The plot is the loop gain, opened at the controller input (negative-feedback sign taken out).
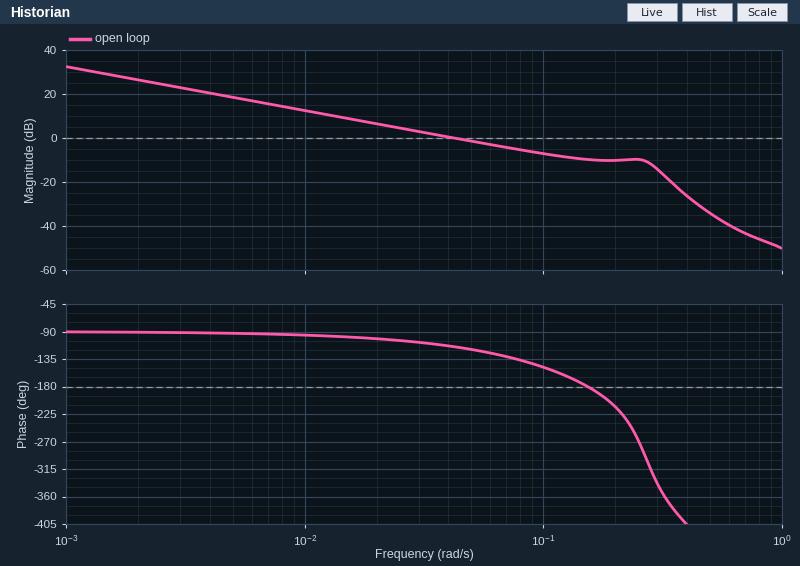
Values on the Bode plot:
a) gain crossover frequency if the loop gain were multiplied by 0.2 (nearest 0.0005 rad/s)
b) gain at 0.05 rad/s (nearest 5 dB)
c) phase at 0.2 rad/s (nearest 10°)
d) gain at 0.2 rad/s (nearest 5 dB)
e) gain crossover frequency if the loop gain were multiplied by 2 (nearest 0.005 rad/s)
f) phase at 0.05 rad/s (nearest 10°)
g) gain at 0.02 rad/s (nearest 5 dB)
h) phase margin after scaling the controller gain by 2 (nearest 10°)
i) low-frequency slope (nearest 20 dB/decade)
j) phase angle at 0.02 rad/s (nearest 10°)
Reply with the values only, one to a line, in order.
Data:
0.0085 rad/s
0 dB
-210°
-10 dB
0.085 rad/s
-120°
5 dB
40°
-20 dB/decade
-100°
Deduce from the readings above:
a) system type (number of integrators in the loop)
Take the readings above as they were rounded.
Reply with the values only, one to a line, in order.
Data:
1
